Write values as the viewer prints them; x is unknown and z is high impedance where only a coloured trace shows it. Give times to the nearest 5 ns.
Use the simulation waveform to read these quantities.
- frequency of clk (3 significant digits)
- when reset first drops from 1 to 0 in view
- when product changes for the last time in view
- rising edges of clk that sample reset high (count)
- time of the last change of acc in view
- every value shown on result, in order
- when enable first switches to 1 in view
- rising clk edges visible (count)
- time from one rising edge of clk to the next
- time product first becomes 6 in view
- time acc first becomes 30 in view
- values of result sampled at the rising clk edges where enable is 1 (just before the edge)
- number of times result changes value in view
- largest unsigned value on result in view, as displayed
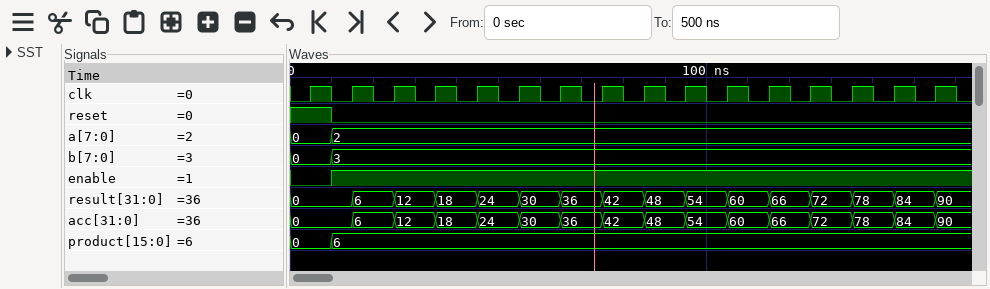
100 MHz
10 ns
10 ns
1
155 ns
0, 6, 12, 18, 24, 30, 36, 42, 48, 54, 60, 66, 72, 78, 84, 90
10 ns
16
10 ns
10 ns
55 ns
0, 6, 12, 18, 24, 30, 36, 42, 48, 54, 60, 66, 72, 78, 84
15
90
